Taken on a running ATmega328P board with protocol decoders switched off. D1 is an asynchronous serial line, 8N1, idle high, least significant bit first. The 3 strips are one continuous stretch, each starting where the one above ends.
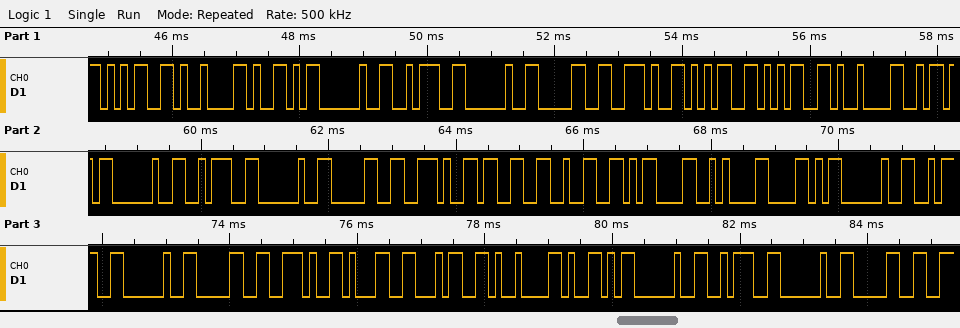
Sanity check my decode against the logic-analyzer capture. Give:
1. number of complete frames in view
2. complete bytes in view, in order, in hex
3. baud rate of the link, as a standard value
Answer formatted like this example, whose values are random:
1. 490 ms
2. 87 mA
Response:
1. 35
2. 0x35 0x09 0x59 0x20 0x3A 0x20 0x30 0x2E 0x35 0x35 0x09 0x5A 0x20 0x3A 0x20 0x30 0x2E 0x33 0x32 0x0D 0x0A 0x58 0x20 0x3A 0x20 0x30 0x2E 0x31 0x34 0x09 0x59 0x20 0x3A 0x20 0x30
3. 9600 baud
